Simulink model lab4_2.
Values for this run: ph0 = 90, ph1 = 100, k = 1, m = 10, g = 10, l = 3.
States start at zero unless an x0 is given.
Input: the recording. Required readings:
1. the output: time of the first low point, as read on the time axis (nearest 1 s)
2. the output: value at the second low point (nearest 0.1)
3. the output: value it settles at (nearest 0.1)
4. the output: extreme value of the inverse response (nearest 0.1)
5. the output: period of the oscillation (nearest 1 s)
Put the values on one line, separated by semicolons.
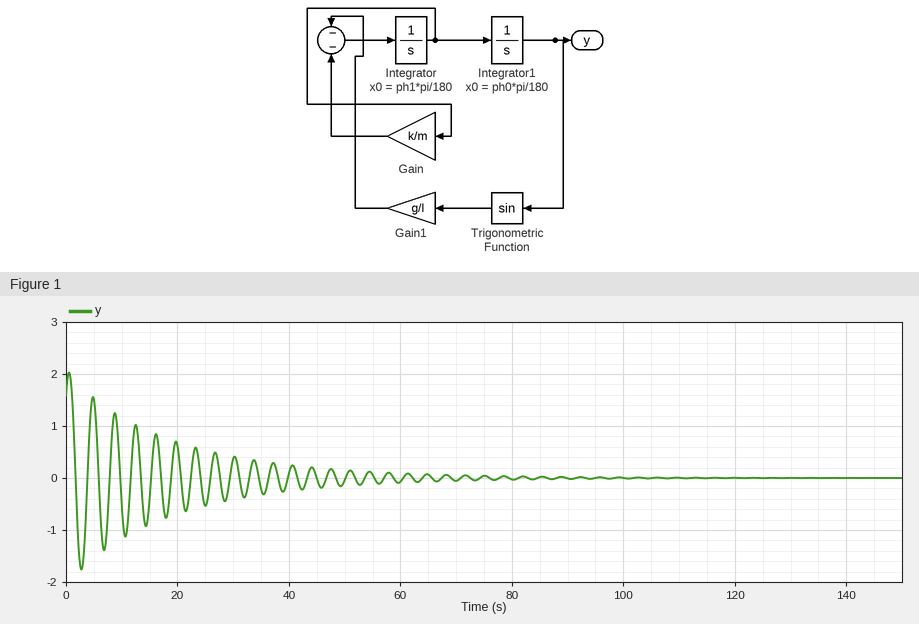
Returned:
3 s; -1.4; 0.0; 2.0; 4 s
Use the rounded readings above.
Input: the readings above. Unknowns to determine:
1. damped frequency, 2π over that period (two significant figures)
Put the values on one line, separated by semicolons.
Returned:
1.6 rad/s
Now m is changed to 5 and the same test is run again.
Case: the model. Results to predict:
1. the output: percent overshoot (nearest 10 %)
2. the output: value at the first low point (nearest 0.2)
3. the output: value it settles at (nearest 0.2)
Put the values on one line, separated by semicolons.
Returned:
100 %; -1.6; 0.0
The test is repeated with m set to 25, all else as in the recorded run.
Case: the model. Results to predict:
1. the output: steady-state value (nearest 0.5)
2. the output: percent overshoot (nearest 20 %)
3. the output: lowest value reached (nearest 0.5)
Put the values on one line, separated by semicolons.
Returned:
0.0; 120 %; -2.0
